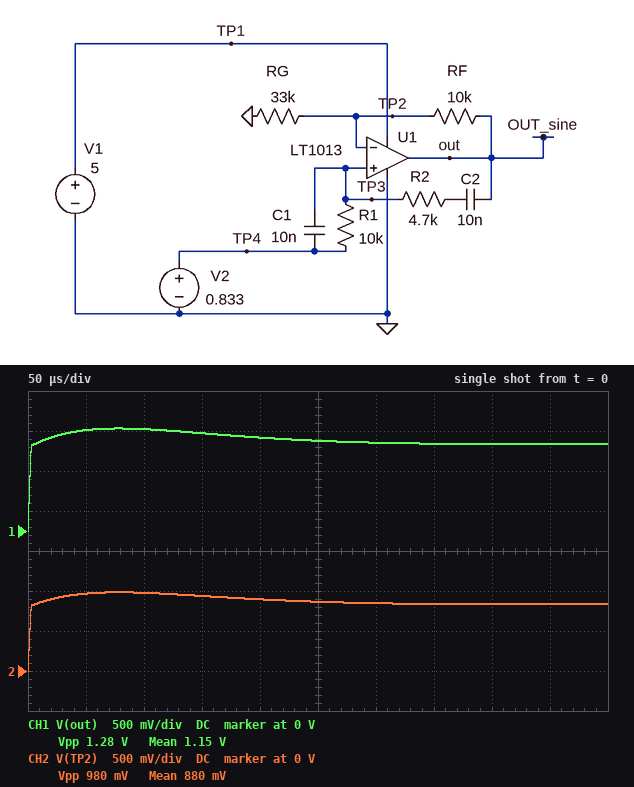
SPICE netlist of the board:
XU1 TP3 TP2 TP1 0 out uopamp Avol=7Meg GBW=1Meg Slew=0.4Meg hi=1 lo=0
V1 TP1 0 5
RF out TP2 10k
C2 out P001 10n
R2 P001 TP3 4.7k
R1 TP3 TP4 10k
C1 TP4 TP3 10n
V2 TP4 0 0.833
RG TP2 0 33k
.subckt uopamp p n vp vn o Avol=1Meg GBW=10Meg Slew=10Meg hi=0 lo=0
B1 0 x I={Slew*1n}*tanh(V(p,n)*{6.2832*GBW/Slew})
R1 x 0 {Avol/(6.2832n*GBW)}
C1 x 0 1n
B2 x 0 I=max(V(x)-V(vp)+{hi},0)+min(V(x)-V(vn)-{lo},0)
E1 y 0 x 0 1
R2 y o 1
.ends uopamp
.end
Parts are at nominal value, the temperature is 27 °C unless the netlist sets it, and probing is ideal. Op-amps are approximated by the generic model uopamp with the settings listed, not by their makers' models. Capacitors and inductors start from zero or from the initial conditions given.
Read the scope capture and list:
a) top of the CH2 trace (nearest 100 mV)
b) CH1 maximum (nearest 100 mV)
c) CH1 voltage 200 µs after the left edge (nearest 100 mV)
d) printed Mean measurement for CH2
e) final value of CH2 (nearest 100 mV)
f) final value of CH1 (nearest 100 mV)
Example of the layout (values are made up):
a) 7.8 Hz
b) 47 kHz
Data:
a) 1.0 V
b) 1.3 V
c) 1.2 V
d) 880 mV
e) 800 mV
f) 1.1 V
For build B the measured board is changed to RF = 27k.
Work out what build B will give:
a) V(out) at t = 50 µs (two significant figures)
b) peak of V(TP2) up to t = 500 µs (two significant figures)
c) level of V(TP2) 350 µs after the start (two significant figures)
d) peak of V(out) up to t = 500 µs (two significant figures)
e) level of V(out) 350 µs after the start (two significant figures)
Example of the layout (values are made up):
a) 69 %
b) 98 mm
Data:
a) 2.3 V
b) 1.4 V
c) 730 mV
d) 2.5 V
e) 1.3 V
